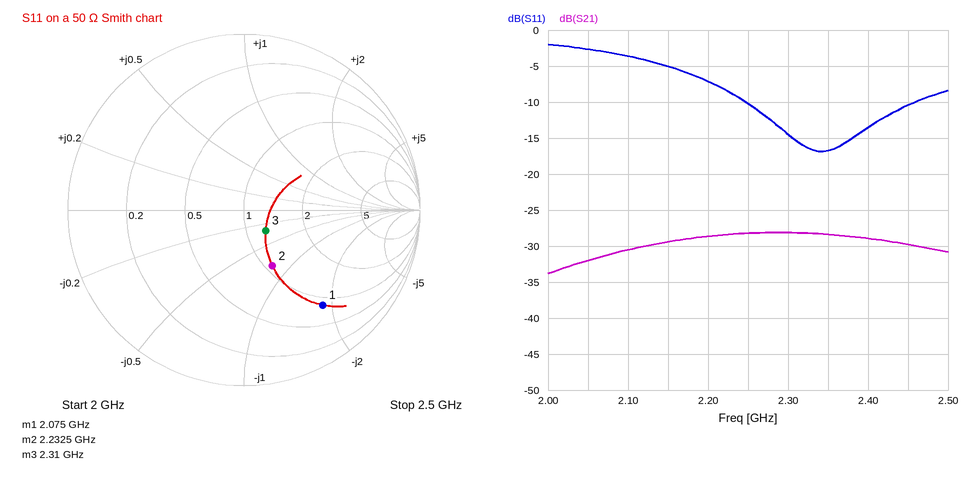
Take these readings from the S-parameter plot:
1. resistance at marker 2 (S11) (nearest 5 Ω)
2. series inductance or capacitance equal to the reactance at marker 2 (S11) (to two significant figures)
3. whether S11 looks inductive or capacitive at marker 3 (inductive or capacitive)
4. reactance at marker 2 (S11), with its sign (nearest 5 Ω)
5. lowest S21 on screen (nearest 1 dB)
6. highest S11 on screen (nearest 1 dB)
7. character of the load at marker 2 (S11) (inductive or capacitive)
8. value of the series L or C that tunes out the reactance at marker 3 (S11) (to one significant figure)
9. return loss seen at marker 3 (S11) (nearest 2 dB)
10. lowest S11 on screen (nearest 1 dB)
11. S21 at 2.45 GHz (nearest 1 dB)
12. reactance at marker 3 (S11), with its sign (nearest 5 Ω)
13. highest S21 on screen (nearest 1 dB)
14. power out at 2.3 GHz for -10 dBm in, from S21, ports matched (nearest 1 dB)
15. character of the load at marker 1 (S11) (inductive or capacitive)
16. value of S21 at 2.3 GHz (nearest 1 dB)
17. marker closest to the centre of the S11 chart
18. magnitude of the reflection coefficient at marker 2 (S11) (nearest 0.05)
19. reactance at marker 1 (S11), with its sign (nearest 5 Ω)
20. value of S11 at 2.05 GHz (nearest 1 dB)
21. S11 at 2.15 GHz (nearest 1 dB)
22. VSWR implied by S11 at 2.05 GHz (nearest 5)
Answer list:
55 Ω
1.8 pF
capacitive
-40 Ω
-34 dB
-2 dB
capacitive
1 nH
16 dB
-17 dB
-30 dB
-15 Ω
-28 dB
-38 dBm
capacitive
-28 dB
marker 3
0.35
-90 Ω
-3 dB
-5 dB
5
